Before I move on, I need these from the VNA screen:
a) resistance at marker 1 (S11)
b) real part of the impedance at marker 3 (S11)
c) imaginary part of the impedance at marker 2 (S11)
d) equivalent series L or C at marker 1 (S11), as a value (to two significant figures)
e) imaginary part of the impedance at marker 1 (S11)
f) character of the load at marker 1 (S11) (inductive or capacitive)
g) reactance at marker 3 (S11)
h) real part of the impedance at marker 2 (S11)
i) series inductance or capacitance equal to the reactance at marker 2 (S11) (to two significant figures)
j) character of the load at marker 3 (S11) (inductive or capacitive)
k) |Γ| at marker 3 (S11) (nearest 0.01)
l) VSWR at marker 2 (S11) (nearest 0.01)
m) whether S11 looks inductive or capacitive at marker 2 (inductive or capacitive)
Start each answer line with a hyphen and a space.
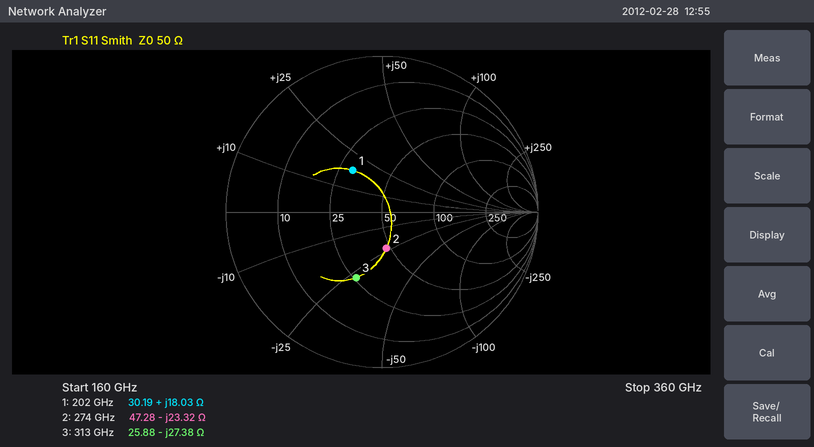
- 30.19 Ω
- 25.88 Ω
- -23.32 Ω
- 14 pH
- +18.03 Ω
- inductive
- -27.38 Ω
- 47.28 Ω
- 25 fF
- capacitive
- 0.45
- 1.61
- capacitive
